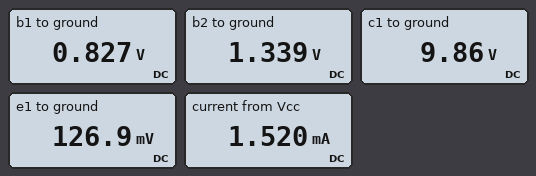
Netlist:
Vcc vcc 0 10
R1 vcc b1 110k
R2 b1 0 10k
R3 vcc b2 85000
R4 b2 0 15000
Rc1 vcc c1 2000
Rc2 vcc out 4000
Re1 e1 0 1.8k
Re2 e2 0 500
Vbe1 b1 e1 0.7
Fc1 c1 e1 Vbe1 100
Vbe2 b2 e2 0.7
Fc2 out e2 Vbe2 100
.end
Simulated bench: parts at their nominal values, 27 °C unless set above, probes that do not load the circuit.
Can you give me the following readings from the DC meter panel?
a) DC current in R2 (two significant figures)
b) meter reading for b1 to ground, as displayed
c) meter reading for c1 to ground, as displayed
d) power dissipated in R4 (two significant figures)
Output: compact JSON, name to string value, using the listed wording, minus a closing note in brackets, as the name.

{"DC current in R2": "83 µA", "meter reading for b1 to ground, as displayed": "0.827 V", "meter reading for c1 to ground, as displayed": "9.86 V", "power dissipated in R4": "120 µW"}
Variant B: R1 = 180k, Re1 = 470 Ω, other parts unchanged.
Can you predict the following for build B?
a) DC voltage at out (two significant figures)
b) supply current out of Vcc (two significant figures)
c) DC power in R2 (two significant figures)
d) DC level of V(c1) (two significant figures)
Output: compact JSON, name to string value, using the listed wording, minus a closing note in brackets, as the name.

{"DC voltage at out": "4.9 V", "supply current out of Vcc": "1.1 mA", "DC power in R2": "31 µW", "DC level of V(c1)": "11 V"}
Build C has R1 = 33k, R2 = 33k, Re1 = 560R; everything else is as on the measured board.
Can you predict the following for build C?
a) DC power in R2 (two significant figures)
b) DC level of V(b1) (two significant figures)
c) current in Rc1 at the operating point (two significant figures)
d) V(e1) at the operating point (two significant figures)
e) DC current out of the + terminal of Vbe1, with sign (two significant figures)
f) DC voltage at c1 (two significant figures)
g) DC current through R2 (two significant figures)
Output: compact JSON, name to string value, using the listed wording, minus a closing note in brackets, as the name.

{"DC power in R2": "490 µW", "DC level of V(b1)": "4.0 V", "current in Rc1 at the operating point": "5.9 mA", "V(e1) at the operating point": "3.3 V", "DC current out of the + terminal of Vbe1, with sign": "-59 µA", "DC voltage at c1": "-1.8 V", "DC current through R2": "120 µA"}
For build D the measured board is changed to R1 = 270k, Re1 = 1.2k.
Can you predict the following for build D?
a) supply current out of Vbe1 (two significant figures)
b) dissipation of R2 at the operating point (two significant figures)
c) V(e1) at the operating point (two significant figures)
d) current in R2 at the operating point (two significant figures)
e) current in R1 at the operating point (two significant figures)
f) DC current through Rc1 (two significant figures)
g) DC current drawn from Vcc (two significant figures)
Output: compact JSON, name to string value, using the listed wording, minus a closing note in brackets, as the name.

{"supply current out of Vbe1": "2.6 µA", "dissipation of R2 at the operating point": "15 µW", "V(e1) at the operating point": "-320 mV", "current in R2 at the operating point": "38 µA", "current in R1 at the operating point": "36 µA", "DC current through Rc1": "260 µA", "DC current drawn from Vcc": "1.1 mA"}
